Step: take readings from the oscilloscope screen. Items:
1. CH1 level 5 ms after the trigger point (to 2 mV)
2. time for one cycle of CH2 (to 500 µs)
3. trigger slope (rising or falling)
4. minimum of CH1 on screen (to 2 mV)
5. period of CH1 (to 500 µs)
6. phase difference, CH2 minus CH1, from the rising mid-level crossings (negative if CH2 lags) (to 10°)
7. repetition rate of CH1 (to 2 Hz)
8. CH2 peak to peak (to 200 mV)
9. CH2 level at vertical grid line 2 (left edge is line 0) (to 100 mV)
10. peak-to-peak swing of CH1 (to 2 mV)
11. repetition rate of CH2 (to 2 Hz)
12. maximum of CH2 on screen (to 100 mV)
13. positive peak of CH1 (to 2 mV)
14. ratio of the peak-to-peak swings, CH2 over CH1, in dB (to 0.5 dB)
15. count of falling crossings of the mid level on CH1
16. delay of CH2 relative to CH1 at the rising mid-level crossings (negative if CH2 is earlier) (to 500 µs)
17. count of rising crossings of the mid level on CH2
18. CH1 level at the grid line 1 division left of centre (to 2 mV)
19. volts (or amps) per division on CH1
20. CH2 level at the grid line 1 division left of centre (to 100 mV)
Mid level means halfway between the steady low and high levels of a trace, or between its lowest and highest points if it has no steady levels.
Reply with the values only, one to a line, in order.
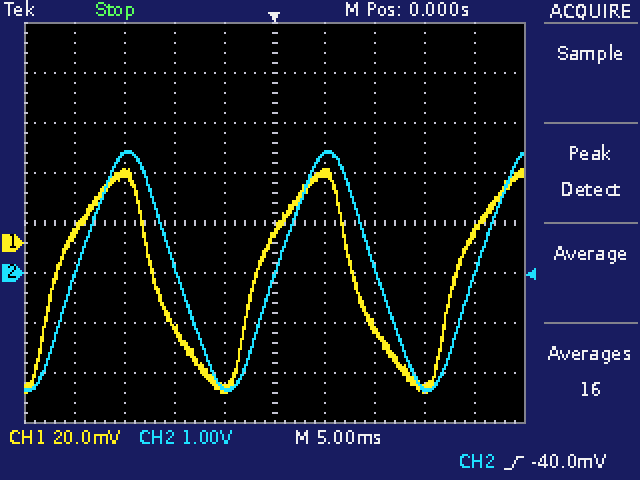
28 mV
20.0 ms
rising
-60 mV
20.0 ms
-40°
50 Hz
4.8 V
2.4 V
90 mV
50 Hz
2.4 V
30 mV
34.5 dB
2
+2.0 ms
3
-58 mV
20 mV
-2.3 V
